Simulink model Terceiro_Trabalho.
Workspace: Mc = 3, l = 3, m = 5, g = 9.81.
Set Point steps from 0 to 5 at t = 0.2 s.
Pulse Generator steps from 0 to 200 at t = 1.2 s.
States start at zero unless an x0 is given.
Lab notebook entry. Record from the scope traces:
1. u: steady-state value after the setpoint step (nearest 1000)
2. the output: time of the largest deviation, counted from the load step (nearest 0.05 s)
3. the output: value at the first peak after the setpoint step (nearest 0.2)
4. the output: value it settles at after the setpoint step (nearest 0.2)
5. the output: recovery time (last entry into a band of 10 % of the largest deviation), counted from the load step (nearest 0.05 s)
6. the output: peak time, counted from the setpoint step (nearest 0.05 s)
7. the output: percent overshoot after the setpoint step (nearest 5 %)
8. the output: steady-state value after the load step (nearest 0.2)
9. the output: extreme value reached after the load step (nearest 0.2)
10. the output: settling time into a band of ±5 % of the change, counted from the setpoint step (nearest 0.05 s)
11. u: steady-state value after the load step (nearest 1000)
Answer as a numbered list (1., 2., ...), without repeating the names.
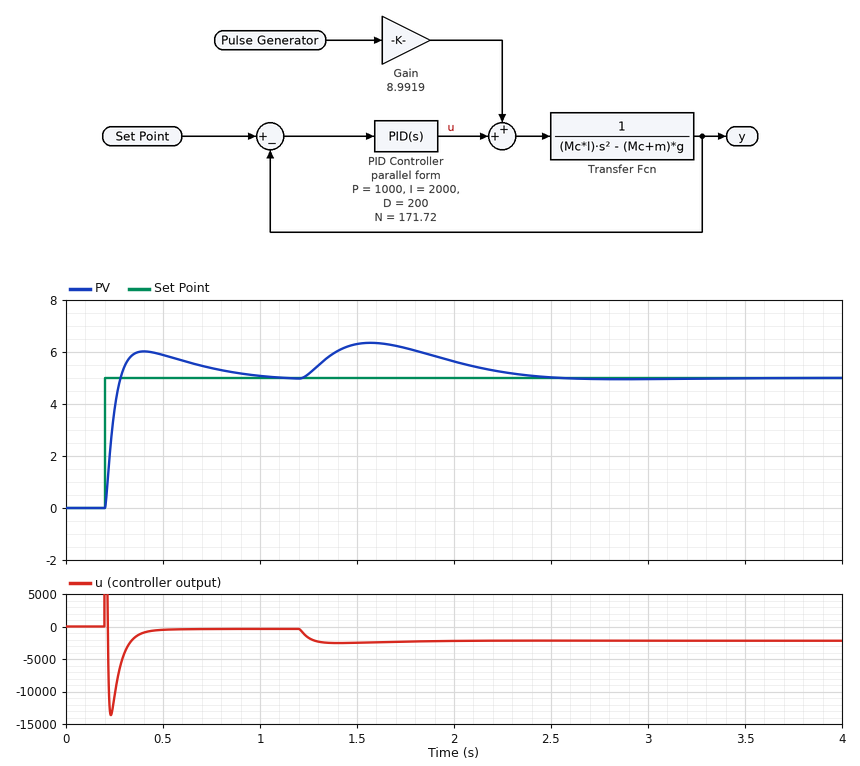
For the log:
1. 0
2. 0.35 s
3. 6.0
4. 5.0
5. 1.15 s
6. 0.20 s
7. 20 %
8. 5.0
9. 6.4
10. 0.65 s
11. -2000
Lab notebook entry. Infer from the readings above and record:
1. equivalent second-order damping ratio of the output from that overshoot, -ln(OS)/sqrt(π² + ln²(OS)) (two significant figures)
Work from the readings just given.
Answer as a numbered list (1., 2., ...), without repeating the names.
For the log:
1. 0.46
